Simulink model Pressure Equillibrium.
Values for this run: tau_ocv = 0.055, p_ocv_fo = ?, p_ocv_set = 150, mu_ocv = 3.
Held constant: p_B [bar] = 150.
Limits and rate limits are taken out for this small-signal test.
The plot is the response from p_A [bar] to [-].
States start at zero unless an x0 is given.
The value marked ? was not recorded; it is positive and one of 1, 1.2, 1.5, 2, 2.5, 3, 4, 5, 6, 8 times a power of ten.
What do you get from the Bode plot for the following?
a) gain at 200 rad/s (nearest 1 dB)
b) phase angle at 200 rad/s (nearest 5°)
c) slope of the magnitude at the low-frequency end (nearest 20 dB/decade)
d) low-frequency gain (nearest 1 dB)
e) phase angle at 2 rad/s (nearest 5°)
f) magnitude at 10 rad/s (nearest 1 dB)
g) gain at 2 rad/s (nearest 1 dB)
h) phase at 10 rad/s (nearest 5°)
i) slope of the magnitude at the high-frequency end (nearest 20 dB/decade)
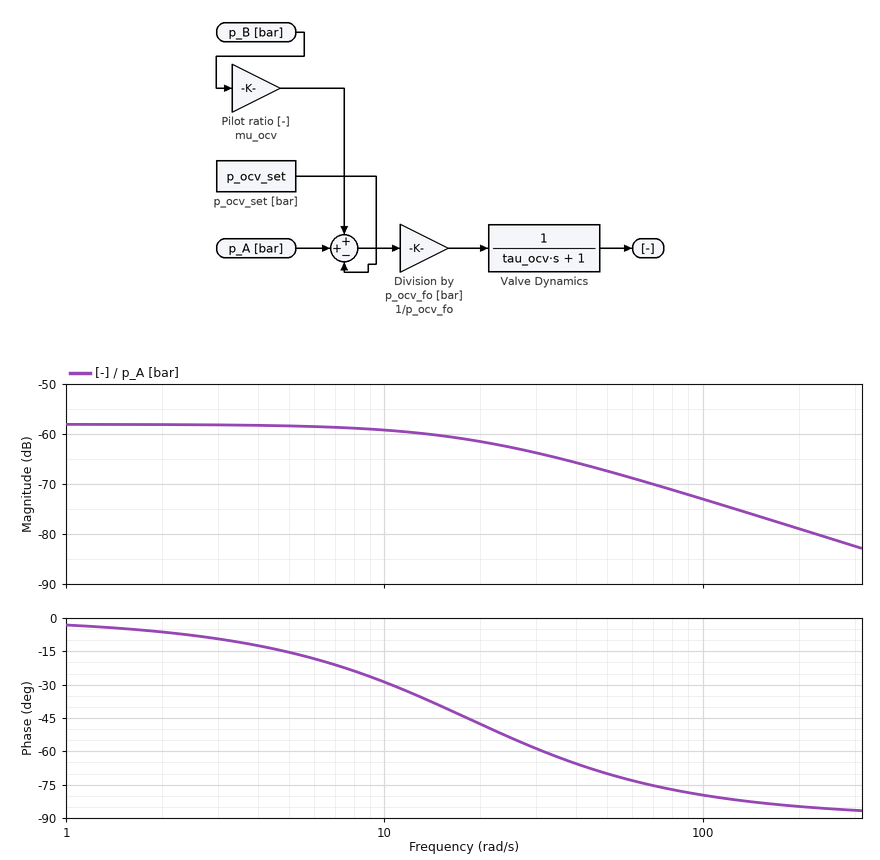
-79 dB
-85°
0 dB/decade
-58 dB
-5°
-59 dB
-58 dB
-30°
-20 dB/decade
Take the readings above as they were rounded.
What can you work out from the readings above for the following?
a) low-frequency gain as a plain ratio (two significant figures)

0.0013
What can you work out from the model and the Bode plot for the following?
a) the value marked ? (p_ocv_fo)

800
